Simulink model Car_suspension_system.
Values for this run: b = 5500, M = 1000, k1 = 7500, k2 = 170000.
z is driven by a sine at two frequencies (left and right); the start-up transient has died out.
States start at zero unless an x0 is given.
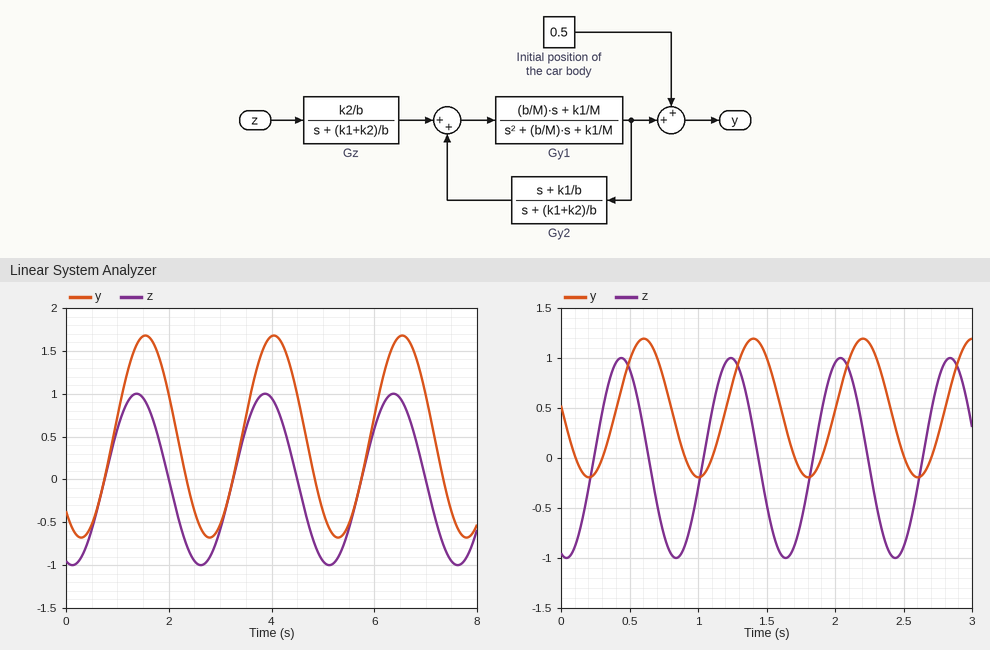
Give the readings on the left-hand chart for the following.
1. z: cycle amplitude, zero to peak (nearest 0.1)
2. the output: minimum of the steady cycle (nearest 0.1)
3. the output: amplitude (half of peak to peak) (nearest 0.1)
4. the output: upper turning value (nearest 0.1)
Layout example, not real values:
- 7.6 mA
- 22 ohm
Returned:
- 1.0
- -0.7
- 1.2
- 1.7
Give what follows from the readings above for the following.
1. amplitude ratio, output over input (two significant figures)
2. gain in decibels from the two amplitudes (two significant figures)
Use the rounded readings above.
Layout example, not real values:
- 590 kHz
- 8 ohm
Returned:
- 1.2
- 1.6 dB
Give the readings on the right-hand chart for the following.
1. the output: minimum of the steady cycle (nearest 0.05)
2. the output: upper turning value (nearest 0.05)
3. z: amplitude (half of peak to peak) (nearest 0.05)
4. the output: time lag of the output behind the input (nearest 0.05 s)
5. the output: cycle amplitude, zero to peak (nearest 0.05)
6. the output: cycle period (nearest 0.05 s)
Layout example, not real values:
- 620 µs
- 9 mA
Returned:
- -0.20
- 1.20
- 1.00
- 0.15 s
- 0.70
- 0.80 s
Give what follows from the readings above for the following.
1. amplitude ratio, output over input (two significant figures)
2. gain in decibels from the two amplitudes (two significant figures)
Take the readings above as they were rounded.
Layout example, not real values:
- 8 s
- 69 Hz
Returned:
- 0.70
- -3.1 dB
